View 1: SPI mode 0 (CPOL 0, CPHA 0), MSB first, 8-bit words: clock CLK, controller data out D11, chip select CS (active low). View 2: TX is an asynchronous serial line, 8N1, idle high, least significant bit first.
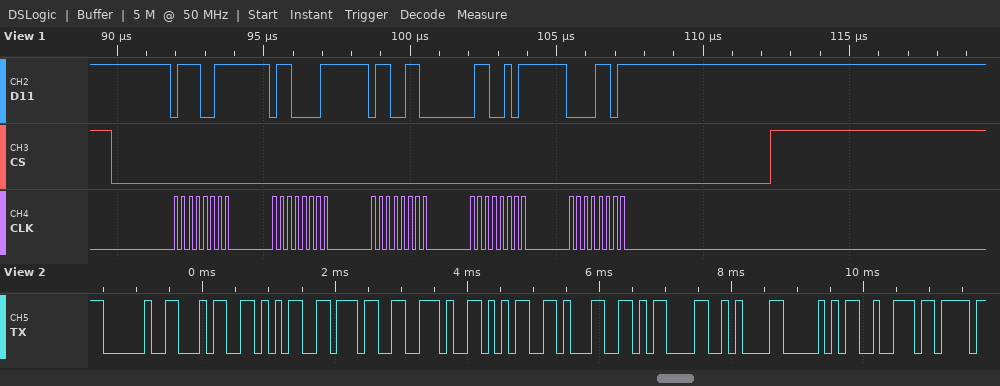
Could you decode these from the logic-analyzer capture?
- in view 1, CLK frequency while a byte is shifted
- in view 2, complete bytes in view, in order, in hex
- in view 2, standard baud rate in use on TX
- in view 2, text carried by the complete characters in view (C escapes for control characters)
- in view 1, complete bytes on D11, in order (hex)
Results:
4 MHz
0x20 0x34 0x35 0x37 0x2E 0x35 0x31 0x0D 0x0A 0x50 0x72
9600 baud
" 457.51\r\nPr"
73 61 66 65 0D
